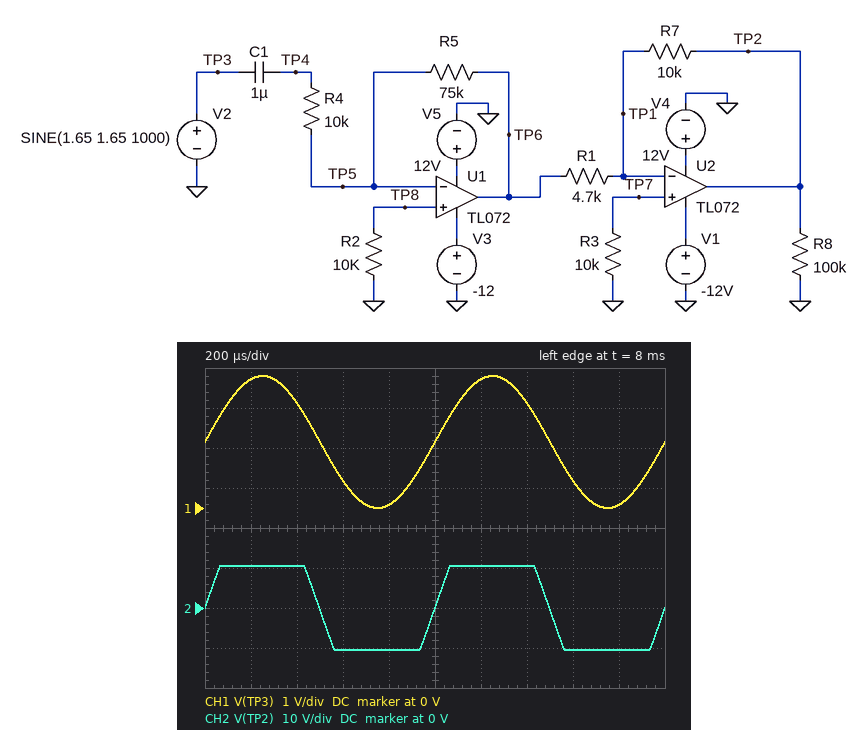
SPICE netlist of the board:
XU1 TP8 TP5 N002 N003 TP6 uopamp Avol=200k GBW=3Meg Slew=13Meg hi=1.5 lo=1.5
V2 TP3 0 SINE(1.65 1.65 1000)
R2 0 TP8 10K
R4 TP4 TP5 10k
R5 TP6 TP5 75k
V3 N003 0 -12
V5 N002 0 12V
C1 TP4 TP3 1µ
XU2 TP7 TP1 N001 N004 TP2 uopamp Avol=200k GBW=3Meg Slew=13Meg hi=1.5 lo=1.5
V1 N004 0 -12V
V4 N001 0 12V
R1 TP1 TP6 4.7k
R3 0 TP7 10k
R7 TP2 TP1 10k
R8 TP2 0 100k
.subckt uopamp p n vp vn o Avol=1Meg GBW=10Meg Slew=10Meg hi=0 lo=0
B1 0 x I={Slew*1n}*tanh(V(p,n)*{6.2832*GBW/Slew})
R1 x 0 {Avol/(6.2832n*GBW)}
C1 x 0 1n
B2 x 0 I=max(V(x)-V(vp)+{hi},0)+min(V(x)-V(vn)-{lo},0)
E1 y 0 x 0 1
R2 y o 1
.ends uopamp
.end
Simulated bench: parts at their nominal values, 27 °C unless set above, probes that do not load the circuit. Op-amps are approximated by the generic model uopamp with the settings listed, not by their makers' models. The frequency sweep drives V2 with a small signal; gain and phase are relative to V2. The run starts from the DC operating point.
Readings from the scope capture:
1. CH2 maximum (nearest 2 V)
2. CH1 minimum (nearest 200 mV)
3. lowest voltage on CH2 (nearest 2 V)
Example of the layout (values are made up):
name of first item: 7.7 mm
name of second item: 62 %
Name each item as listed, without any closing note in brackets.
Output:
CH2 maximum: 10 V
CH1 minimum: 0 V
lowest voltage on CH2: -10 V
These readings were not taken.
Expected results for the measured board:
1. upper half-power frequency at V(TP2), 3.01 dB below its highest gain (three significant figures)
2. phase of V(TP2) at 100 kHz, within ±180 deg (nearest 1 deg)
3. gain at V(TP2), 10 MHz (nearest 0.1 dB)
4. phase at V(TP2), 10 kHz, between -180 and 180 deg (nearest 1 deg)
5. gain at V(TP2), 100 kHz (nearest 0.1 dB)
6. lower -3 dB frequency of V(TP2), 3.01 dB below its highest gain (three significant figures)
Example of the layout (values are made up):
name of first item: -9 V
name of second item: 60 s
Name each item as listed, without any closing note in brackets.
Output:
upper half-power frequency at V(TP2), 3.01 dB below its highest gain: 316 kHz
phase of V(TP2) at 100 kHz, within ±180 deg: -22 deg
gain at V(TP2), 10 MHz: -25.4 dB
phase at V(TP2), 10 kHz, between -180 and 180 deg: -2 deg
gain at V(TP2), 100 kHz: 23.7 dB
lower -3 dB frequency of V(TP2), 3.01 dB below its highest gain: 15.9 Hz
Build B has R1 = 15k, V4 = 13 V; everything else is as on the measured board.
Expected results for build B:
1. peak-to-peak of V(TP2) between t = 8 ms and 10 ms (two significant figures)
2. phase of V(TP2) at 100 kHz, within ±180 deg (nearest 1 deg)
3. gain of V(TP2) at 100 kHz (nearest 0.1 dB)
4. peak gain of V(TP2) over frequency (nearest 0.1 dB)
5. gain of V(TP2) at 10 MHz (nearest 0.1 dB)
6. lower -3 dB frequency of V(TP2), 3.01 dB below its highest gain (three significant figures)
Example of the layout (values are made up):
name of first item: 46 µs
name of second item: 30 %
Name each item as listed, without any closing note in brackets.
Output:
peak-to-peak of V(TP2) between t = 8 ms and 10 ms: 14 V
phase of V(TP2) at 100 kHz, within ±180 deg: -19 deg
gain of V(TP2) at 100 kHz: 13.6 dB
peak gain of V(TP2) over frequency: 14.0 dB
gain of V(TP2) at 10 MHz: -30.1 dB
lower -3 dB frequency of V(TP2), 3.01 dB below its highest gain: 15.9 Hz
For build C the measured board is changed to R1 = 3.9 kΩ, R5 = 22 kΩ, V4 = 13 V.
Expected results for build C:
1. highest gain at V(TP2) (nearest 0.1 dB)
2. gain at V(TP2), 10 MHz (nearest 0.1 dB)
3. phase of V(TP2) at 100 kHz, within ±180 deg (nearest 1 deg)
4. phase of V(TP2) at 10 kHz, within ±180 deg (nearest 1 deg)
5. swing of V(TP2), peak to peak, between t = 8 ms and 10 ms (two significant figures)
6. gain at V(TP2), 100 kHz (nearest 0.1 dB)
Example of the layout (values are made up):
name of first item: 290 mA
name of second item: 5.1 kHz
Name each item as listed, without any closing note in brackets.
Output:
highest gain at V(TP2): 15.0 dB
gain at V(TP2), 10 MHz: -27.1 dB
phase of V(TP2) at 100 kHz, within ±180 deg: -13 deg
phase of V(TP2) at 10 kHz, within ±180 deg: -1 deg
swing of V(TP2), peak to peak, between t = 8 ms and 10 ms: 19 V
gain at V(TP2), 100 kHz: 14.9 dB
